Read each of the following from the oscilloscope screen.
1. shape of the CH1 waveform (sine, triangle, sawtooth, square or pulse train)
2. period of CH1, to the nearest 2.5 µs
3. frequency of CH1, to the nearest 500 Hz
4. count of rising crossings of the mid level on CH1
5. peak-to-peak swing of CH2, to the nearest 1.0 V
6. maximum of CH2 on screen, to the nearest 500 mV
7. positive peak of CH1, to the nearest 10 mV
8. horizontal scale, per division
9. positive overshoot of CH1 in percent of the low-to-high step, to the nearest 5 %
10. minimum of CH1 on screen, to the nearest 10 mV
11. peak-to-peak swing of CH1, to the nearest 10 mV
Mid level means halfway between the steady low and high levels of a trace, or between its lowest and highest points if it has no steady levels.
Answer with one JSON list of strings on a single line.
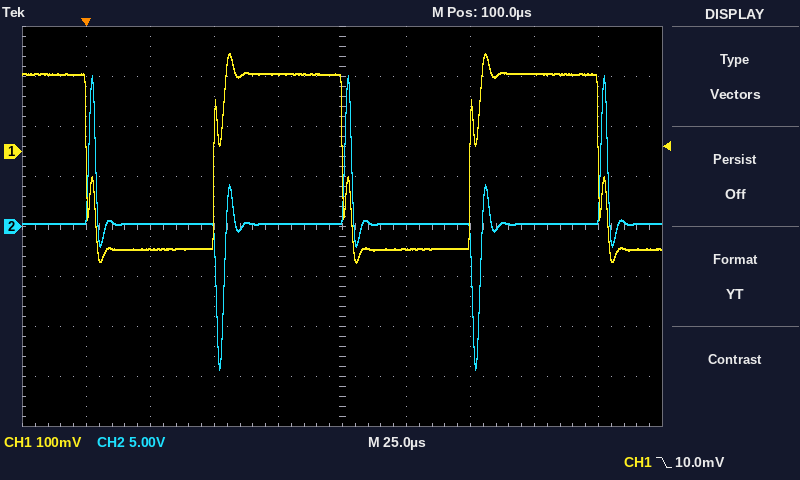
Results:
["square", "100.0 µs", "10.0 kHz", "2", "29.0 V", "15.0 V", "200 mV", "25 µs", "10 %", "-220 mV", "420 mV"]
